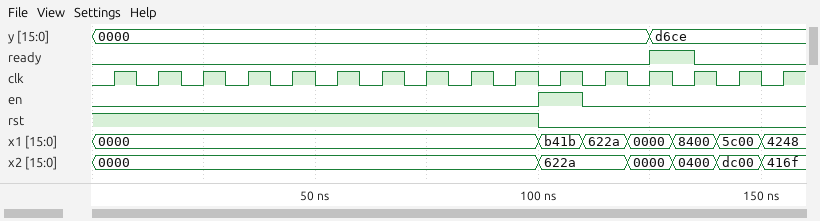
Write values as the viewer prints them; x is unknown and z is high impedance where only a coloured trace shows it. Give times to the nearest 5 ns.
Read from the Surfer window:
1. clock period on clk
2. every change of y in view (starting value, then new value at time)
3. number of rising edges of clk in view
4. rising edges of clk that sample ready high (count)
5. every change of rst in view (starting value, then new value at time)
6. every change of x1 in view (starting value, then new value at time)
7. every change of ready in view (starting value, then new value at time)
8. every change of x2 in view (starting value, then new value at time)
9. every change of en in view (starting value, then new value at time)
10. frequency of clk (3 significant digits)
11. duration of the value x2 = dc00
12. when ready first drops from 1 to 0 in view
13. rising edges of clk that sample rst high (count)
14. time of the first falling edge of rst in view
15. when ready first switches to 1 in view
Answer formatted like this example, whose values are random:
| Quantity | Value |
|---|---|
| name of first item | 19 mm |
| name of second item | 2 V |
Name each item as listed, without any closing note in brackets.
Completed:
| Quantity | Value |
|---|---|
| clock period on clk | 10 ns |
| every change of y in view | 0000, d6ce at 125 ns |
| number of rising edges of clk in view | 16 |
| rising edges of clk that sample ready high | 1 |
| every change of rst in view | 1, 0 at 100 ns |
| every change of x1 in view | 0000, b41b at 100 ns, 622a at 110 ns, 0000 at 120 ns, 8400 at 130 ns, 5c00 at 140 ns, 4248 at 150 ns |
| every change of ready in view | 0, 1 at 125 ns, 0 at 135 ns |
| every change of x2 in view | 0000, 622a at 100 ns, 0000 at 120 ns, 0400 at 130 ns, dc00 at 140 ns, 416f at 150 ns |
| every change of en in view | 0, 1 at 100 ns, 0 at 110 ns |
| frequency of clk | 100 MHz |
| duration of the value x2 = dc00 | 10 ns |
| when ready first drops from 1 to 0 in view | 135 ns |
| rising edges of clk that sample rst high | 10 |
| time of the first falling edge of rst in view | 100 ns |
| when ready first switches to 1 in view | 125 ns |
